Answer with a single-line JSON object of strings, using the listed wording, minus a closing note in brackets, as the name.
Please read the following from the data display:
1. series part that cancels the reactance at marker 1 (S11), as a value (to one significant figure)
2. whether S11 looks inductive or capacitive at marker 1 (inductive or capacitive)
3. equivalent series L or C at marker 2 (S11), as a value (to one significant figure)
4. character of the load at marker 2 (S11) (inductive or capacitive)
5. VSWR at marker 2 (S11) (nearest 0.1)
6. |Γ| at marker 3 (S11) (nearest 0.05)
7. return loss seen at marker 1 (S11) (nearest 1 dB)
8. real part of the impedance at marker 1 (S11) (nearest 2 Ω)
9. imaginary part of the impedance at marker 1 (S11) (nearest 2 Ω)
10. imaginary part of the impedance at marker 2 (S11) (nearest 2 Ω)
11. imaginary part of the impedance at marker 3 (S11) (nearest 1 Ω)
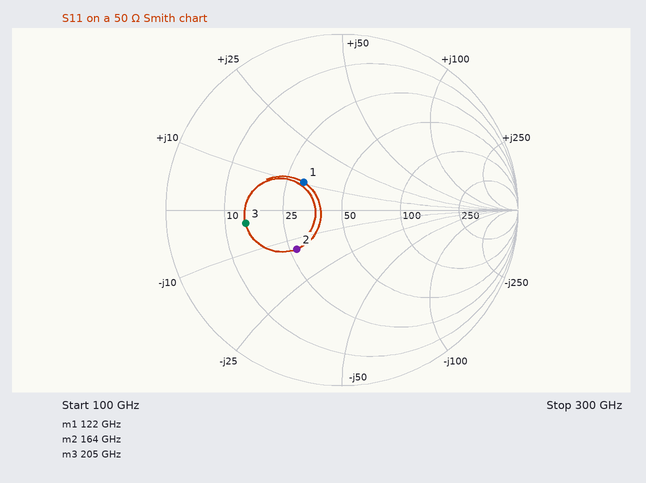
{"series part that cancels the reactance at marker 1 (S11), as a value": "100 fF", "whether S11 looks inductive or capacitive at marker 1": "inductive", "equivalent series L or C at marker 2 (S11), as a value": "70 fF", "character of the load at marker 2 (S11)": "capacitive", "VSWR at marker 2 (S11)": "2.0", "|Γ| at marker 3 (S11)": "0.55", "return loss seen at marker 1 (S11)": "11 dB", "real part of the impedance at marker 1 (S11)": "30 Ω", "imaginary part of the impedance at marker 1 (S11)": "+10 Ω", "imaginary part of the impedance at marker 2 (S11)": "-14 Ω", "imaginary part of the impedance at marker 3 (S11)": "-3 Ω"}
